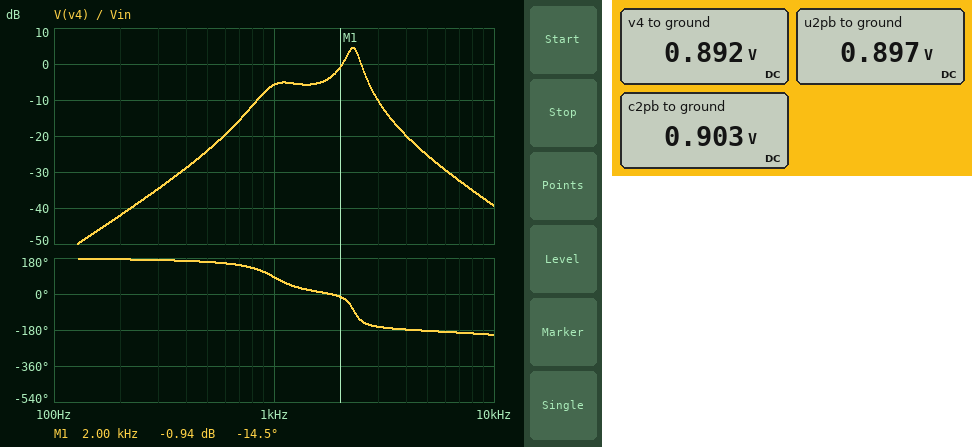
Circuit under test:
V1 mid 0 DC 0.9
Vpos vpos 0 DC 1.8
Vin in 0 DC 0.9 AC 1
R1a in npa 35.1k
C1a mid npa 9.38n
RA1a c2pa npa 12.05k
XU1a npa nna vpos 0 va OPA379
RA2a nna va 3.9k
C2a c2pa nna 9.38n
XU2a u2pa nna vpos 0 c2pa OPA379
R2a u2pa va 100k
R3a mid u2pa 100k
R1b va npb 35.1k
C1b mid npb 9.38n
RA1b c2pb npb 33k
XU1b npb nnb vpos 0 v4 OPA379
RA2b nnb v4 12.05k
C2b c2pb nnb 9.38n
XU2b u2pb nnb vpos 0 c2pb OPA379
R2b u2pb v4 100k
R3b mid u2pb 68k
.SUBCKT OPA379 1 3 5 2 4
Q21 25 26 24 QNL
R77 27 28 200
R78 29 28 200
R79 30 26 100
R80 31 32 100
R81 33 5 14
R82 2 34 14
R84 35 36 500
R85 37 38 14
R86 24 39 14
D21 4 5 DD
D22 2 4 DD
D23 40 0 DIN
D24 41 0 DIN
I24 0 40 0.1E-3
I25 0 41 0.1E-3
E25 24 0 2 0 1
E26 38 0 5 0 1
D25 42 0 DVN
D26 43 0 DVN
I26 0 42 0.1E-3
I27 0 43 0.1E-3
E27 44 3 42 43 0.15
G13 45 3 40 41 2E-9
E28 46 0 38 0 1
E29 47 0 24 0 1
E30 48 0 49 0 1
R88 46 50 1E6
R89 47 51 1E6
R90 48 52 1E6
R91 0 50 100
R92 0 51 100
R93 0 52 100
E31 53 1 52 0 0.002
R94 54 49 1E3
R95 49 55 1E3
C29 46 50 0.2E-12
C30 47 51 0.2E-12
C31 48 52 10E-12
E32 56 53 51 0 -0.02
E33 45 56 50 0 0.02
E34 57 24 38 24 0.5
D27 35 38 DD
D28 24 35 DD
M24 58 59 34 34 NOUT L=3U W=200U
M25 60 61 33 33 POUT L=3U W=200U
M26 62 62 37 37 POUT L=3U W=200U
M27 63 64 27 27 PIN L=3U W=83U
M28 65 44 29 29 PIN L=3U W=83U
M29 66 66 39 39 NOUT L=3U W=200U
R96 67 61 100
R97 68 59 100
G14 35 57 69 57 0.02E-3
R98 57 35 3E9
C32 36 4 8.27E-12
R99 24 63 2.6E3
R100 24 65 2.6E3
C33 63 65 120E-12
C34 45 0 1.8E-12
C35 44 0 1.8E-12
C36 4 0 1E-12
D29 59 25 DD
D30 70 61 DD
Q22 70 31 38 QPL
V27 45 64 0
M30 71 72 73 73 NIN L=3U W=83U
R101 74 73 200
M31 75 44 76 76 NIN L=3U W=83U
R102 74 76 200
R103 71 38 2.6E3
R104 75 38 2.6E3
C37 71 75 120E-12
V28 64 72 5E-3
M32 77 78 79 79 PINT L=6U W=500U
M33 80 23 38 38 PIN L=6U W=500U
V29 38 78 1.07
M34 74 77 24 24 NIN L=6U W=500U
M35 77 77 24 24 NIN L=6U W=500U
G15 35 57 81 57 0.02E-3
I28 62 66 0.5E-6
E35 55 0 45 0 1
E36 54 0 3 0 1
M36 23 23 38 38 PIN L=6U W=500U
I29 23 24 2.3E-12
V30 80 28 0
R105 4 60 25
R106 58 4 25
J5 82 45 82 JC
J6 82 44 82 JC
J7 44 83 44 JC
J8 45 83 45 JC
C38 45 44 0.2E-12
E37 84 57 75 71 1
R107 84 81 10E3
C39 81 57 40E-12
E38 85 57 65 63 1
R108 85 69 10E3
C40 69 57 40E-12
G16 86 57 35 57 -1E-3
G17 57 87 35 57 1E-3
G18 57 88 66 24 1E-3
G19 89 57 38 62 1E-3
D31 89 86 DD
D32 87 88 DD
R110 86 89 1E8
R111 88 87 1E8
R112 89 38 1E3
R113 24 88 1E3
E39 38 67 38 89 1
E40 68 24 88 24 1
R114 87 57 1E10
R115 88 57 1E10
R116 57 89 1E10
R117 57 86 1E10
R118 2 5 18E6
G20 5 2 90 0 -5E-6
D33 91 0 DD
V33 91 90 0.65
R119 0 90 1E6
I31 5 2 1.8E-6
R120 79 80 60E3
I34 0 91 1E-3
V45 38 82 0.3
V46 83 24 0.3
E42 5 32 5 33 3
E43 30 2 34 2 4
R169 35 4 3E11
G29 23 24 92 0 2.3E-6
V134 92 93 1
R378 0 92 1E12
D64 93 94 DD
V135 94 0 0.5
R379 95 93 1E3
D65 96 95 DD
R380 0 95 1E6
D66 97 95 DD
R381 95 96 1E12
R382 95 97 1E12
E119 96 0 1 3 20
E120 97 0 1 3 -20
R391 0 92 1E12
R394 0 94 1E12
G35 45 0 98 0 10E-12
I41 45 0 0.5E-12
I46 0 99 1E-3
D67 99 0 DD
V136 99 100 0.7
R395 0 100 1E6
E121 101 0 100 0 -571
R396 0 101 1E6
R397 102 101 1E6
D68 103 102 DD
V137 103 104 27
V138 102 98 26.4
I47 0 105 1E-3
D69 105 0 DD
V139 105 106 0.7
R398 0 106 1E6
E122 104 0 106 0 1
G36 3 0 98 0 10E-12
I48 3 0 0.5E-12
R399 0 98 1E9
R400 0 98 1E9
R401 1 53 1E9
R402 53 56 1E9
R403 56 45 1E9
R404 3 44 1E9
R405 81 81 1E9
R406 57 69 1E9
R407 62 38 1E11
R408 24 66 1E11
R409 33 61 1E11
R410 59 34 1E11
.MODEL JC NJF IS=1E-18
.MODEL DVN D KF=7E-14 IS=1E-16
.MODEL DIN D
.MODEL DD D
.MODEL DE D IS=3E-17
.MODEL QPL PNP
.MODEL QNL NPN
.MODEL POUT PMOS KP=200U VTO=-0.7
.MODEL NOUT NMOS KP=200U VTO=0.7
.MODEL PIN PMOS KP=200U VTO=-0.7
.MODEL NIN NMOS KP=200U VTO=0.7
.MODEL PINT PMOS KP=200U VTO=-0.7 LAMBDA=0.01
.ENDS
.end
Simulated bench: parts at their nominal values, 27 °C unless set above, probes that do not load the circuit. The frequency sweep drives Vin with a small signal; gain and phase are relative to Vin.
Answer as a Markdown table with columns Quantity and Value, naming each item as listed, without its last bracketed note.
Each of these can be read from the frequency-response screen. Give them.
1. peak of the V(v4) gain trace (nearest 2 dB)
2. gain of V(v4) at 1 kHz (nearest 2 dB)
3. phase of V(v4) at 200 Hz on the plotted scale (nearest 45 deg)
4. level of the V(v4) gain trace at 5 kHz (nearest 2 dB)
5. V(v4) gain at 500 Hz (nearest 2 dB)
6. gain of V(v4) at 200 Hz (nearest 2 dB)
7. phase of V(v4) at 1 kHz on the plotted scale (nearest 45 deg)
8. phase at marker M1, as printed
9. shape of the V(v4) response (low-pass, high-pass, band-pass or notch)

| Quantity | Value |
|---|---|
| peak of the V(v4) gain trace | 4 dB |
| gain of V(v4) at 1 kHz | -6 dB |
| phase of V(v4) at 200 Hz on the plotted scale | 180 deg |
| level of the V(v4) gain trace at 5 kHz | -26 dB |
| V(v4) gain at 500 Hz | -24 dB |
| gain of V(v4) at 200 Hz | -42 dB |
| phase of V(v4) at 1 kHz on the plotted scale | 90 deg |
| phase at marker M1, as printed | -14.5 deg |
| shape of the V(v4) response | band-pass |
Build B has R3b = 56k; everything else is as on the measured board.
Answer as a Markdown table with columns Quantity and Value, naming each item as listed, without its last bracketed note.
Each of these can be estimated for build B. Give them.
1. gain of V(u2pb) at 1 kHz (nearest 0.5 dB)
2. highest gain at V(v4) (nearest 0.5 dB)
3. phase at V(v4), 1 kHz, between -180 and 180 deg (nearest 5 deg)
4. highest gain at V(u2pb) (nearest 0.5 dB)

| Quantity | Value |
|---|---|
| gain of V(u2pb) at 1 kHz | -14.5 dB |
| highest gain at V(v4) | 6.0 dB |
| phase at V(v4), 1 kHz, between -180 and 180 deg | 110 deg |
| highest gain at V(u2pb) | -3.0 dB |
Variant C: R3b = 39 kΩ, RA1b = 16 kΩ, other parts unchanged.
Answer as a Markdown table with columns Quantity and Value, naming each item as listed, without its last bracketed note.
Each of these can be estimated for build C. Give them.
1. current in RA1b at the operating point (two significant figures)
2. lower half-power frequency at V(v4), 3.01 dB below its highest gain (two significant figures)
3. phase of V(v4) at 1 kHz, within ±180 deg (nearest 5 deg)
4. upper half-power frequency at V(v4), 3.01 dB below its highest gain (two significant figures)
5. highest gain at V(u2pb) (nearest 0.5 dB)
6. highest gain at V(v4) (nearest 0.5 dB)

| Quantity | Value |
|---|---|
| current in RA1b at the operating point | 230 nA |
| lower half-power frequency at V(v4), 3.01 dB below its highest gain | 1.8 kHz |
| phase of V(v4) at 1 kHz, within ±180 deg | 165 deg |
| upper half-power frequency at V(v4), 3.01 dB below its highest gain | 2.4 kHz |
| highest gain at V(u2pb) | 3.5 dB |
| highest gain at V(v4) | 14.5 dB |
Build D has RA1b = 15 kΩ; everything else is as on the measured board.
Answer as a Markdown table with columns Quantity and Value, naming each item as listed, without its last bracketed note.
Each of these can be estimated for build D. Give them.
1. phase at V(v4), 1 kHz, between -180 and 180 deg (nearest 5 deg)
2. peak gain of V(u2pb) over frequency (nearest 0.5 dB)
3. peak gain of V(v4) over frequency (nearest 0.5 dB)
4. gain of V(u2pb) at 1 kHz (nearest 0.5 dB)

| Quantity | Value |
|---|---|
| phase at V(v4), 1 kHz, between -180 and 180 deg | 155 deg |
| peak gain of V(u2pb) over frequency | -1.0 dB |
| peak gain of V(v4) over frequency | 7.0 dB |
| gain of V(u2pb) at 1 kHz | -22.5 dB |
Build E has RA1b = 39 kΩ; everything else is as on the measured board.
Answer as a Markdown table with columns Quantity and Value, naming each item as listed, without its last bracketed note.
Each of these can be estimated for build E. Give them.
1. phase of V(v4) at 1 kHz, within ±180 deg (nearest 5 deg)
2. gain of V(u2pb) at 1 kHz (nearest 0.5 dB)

| Quantity | Value |
|---|---|
| phase of V(v4) at 1 kHz, within ±180 deg | 65 deg |
| gain of V(u2pb) at 1 kHz | -14.0 dB |
